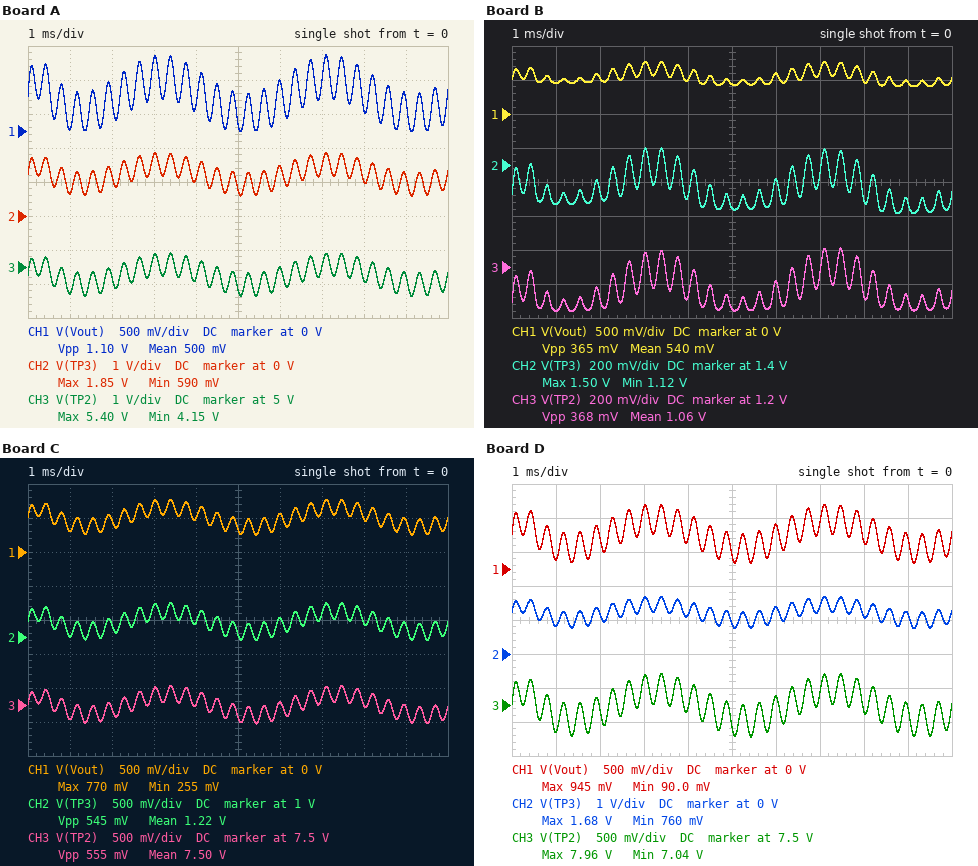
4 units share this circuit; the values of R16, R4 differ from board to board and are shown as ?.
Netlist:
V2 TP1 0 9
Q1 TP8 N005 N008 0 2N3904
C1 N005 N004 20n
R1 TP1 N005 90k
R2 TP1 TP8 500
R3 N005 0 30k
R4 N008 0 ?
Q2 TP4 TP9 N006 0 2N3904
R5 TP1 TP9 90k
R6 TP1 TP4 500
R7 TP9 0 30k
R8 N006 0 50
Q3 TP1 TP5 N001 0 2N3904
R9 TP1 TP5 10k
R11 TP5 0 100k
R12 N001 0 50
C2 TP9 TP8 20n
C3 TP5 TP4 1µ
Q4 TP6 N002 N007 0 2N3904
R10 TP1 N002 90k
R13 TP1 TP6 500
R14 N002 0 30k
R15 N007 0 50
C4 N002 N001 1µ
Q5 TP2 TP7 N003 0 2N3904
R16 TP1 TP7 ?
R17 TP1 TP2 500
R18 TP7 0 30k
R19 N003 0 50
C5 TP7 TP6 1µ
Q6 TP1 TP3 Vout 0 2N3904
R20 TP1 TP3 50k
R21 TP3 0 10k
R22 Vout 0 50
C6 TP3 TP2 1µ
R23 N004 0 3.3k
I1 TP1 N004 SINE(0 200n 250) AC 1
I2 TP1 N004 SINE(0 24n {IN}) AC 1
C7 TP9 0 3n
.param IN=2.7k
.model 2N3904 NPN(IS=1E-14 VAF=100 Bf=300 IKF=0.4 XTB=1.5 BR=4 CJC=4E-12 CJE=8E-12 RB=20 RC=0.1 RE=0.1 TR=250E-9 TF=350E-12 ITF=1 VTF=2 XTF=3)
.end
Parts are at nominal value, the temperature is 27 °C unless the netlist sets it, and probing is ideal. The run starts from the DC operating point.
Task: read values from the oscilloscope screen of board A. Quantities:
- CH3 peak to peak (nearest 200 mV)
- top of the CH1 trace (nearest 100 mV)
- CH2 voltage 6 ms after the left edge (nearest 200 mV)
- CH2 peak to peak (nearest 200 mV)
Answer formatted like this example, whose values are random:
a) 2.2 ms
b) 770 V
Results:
a) 1.2 V
b) 1.1 V
c) 1.4 V
d) 1.2 V
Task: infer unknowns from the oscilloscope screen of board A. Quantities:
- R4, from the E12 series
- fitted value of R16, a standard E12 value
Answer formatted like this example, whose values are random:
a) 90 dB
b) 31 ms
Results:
a) 39 Ω
b) 120 kΩ
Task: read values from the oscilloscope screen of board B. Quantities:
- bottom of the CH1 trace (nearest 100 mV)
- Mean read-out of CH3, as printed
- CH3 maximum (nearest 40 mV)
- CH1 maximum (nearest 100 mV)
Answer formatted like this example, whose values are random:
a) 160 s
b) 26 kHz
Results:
a) 400 mV
b) 1.06 V
c) 1.32 V
d) 800 mV
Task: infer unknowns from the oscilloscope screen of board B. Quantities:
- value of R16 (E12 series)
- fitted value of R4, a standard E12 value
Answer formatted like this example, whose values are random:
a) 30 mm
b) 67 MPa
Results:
a) 68 kΩ
b) 150 Ω
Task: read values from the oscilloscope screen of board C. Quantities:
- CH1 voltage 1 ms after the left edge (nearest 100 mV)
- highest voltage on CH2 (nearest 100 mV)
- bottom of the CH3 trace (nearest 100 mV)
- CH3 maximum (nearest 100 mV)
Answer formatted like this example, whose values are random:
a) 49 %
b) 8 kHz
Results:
a) 300 mV
b) 1.5 V
c) 7.2 V
d) 7.8 V
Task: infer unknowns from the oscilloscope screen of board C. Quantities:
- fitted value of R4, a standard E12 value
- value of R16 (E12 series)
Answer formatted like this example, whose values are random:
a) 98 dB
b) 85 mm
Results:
a) 120 Ω
b) 220 kΩ
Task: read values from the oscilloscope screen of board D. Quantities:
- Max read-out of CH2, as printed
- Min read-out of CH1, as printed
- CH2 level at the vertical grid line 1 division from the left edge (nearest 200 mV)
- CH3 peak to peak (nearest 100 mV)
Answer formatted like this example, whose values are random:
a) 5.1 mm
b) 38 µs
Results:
a) 1.68 V
b) 90.0 mV
c) 800 mV
d) 900 mV
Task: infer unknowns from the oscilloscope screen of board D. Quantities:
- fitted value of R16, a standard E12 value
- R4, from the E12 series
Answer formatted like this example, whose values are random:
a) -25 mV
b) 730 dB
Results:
a) 220 kΩ
b) 56 Ω
